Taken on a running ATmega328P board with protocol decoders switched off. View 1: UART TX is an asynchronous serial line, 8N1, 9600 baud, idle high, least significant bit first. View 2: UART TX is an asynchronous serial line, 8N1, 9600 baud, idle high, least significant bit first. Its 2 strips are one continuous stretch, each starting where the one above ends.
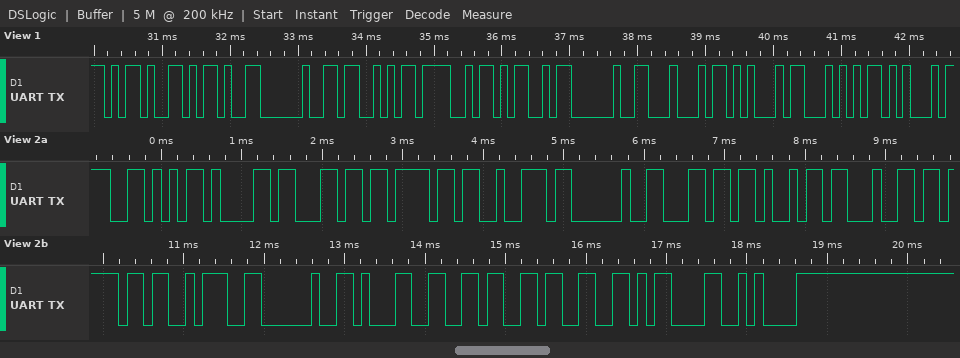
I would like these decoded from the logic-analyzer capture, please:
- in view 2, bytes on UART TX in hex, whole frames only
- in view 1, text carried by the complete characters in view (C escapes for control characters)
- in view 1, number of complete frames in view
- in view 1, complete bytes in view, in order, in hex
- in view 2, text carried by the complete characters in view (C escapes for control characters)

56 61 6C 6F 72 20 6C 69 64 6F 3A 20 31 36 33 0D 0A
"-- SOM DETE"
11
2D 2D 20 53 4F 4D 20 44 45 54 45
"Valor lido: 163\r\n"
